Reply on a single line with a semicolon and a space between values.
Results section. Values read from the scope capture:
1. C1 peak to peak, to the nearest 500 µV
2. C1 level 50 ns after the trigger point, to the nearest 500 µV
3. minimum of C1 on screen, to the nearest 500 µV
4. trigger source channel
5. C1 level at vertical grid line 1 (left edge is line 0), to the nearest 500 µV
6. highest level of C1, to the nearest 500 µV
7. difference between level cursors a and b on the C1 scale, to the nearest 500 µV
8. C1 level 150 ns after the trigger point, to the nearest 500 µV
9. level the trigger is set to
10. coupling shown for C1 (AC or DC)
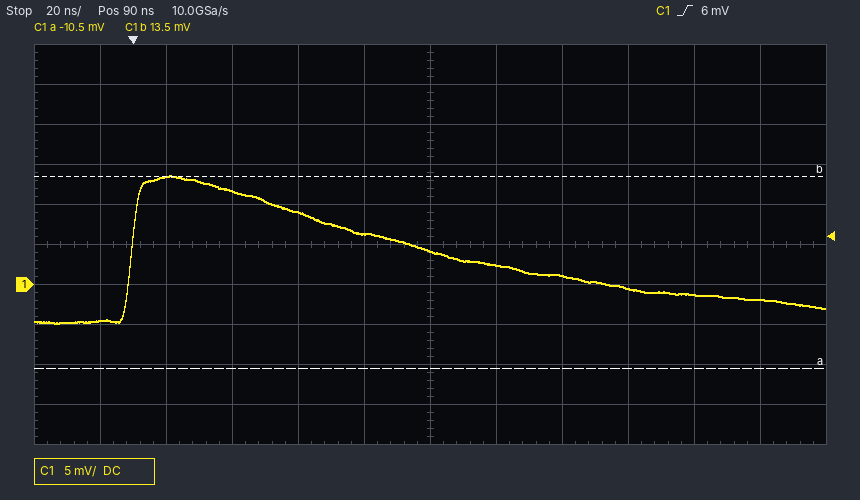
18.5 mV; 9.0 mV; -5.0 mV; C1; -4.5 mV; 13.5 mV; 24.0 mV; -500 µV; 6 mV; DC
